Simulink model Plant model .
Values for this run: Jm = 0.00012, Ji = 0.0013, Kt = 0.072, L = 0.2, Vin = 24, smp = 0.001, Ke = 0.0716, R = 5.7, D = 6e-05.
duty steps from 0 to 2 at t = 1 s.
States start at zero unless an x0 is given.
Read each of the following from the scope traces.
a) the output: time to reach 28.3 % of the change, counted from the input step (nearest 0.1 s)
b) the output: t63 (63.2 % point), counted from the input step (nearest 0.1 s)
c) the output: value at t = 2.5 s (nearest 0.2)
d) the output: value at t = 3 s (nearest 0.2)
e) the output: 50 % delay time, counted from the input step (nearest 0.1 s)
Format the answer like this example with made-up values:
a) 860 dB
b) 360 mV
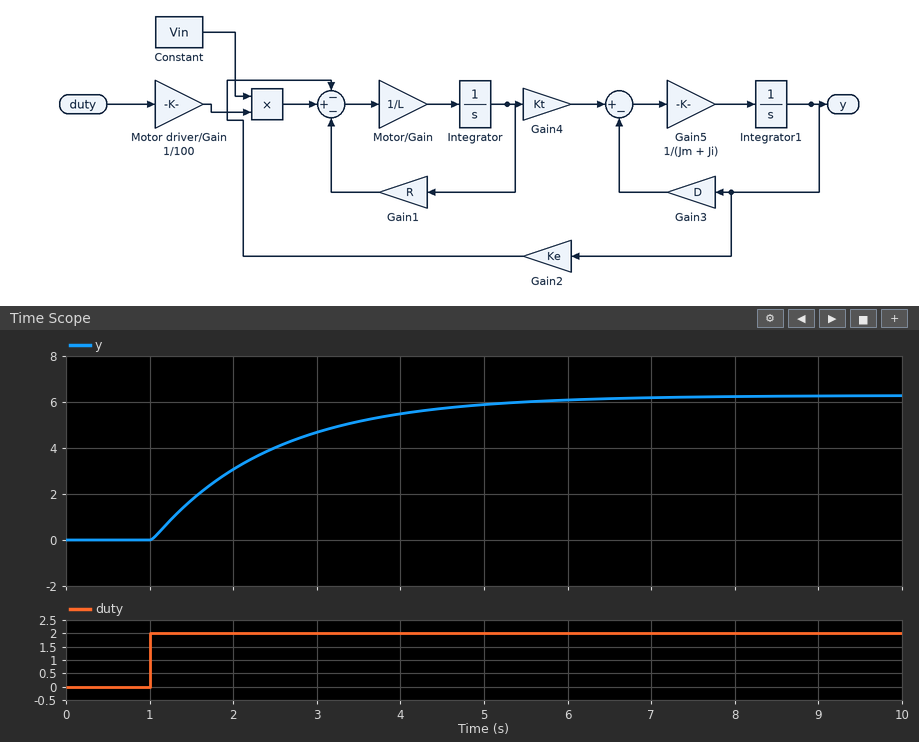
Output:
a) 0.5 s
b) 1.5 s
c) 4.0
d) 4.6
e) 1.0 s
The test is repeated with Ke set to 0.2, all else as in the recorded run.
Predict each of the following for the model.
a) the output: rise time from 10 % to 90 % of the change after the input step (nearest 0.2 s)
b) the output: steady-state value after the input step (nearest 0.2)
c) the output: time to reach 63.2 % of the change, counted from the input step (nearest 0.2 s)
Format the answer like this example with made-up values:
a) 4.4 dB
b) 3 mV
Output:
a) 1.2 s
b) 2.4
c) 0.6 s
